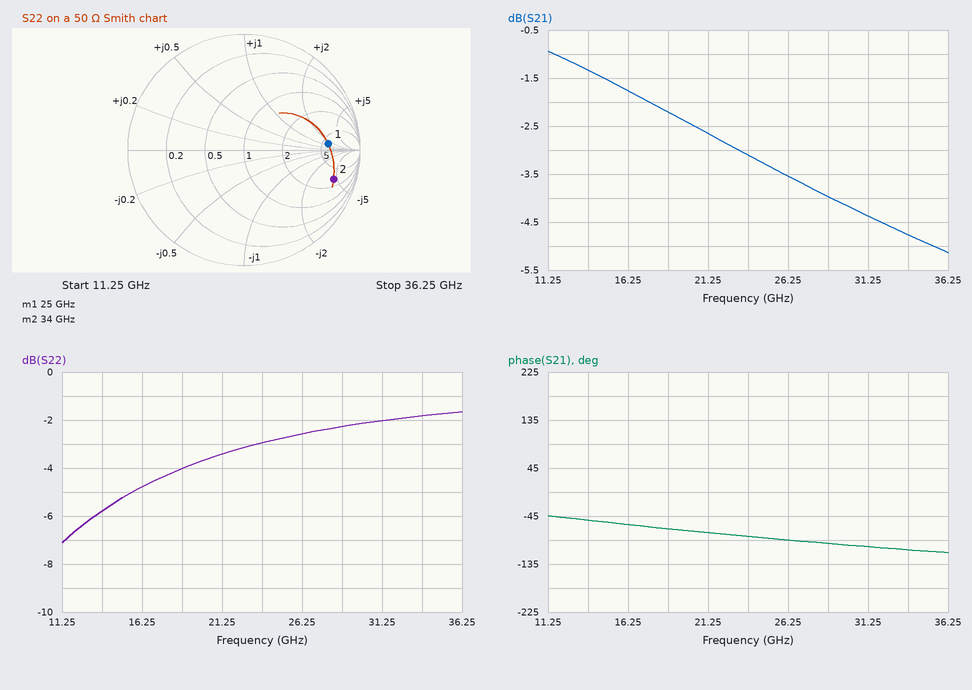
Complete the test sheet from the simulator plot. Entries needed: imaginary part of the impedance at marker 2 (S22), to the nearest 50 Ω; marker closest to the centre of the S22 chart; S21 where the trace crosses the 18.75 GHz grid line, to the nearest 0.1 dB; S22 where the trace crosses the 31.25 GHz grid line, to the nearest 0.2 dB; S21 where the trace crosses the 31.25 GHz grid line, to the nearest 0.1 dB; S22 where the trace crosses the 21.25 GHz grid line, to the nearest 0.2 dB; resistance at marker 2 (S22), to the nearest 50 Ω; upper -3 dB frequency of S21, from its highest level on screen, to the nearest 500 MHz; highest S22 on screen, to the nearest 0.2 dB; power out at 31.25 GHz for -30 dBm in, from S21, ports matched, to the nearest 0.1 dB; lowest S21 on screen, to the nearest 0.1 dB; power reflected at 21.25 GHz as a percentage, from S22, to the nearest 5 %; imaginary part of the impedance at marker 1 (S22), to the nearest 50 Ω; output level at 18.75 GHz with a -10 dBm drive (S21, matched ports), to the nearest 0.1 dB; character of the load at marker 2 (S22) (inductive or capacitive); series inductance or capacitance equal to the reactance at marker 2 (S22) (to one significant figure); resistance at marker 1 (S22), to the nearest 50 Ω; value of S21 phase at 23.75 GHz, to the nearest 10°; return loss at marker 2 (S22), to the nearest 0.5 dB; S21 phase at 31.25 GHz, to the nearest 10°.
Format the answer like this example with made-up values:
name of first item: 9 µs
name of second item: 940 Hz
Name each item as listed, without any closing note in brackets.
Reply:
imaginary part of the impedance at marker 2 (S22), to the nearest 50 Ω: -200 Ω
marker closest to the centre of the S22 chart: marker 1
S21 where the trace crosses the 18.75 GHz grid line, to the nearest 0.1 dB: -2.2 dB
S22 where the trace crosses the 31.25 GHz grid line, to the nearest 0.2 dB: -2.0 dB
S21 where the trace crosses the 31.25 GHz grid line, to the nearest 0.1 dB: -4.4 dB
S22 where the trace crosses the 21.25 GHz grid line, to the nearest 0.2 dB: -3.4 dB
resistance at marker 2 (S22), to the nearest 50 Ω: 150 Ω
upper -3 dB frequency of S21, from its highest level on screen, to the nearest 500 MHz: 28.5 GHz
highest S22 on screen, to the nearest 0.2 dB: -1.6 dB
power out at 31.25 GHz for -30 dBm in, from S21, ports matched, to the nearest 0.1 dB: -34.4 dBm
lowest S21 on screen, to the nearest 0.1 dB: -5.1 dB
power reflected at 21.25 GHz as a percentage, from S22, to the nearest 5 %: 45 %
imaginary part of the impedance at marker 1 (S22), to the nearest 50 Ω: +50 Ω
output level at 18.75 GHz with a -10 dBm drive (S21, matched ports), to the nearest 0.1 dB: -12.2 dBm
character of the load at marker 2 (S22): capacitive
series inductance or capacitance equal to the reactance at marker 2 (S22): 20 fF
resistance at marker 1 (S22), to the nearest 50 Ω: 300 Ω
value of S21 phase at 23.75 GHz, to the nearest 10°: -80°
return loss at marker 2 (S22), to the nearest 0.5 dB: 2.0 dB
S21 phase at 31.25 GHz, to the nearest 10°: -100°
